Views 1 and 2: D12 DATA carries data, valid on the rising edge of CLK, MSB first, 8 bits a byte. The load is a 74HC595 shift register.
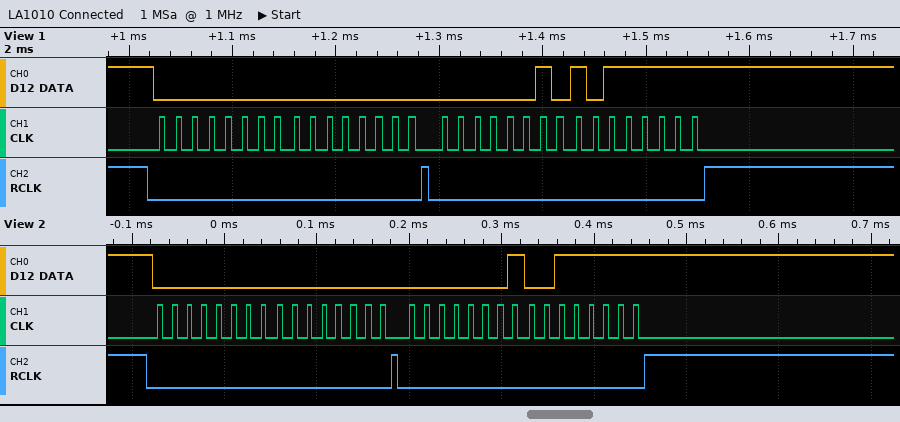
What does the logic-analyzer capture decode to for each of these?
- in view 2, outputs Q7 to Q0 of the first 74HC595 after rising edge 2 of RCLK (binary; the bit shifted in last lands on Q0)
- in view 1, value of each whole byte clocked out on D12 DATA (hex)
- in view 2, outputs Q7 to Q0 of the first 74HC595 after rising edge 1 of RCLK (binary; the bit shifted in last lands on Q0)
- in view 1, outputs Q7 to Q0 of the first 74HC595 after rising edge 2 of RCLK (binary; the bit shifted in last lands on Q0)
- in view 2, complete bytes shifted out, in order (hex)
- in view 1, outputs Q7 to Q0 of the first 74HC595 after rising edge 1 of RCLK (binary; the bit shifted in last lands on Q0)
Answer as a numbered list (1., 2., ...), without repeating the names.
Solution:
1. 00111111
2. 0x00 0x00 0x02 0xBF
3. 00000000
4. 10111111
5. 00 00 01 3F
6. 00000000
